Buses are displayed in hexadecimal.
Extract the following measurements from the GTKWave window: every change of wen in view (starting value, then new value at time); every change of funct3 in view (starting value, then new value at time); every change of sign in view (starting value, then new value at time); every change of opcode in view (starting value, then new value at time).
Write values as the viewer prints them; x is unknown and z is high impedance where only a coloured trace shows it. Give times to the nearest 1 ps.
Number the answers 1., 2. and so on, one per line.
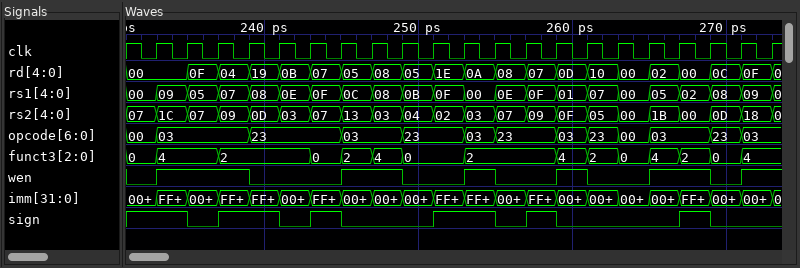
1. 0, 1 at 233 ps, 0 at 239 ps, 1 at 245 ps, 0 at 249 ps, 1 at 253 ps, 0 at 255 ps, 1 at 259 ps, 0 at 261 ps, 1 at 265 ps, 0 at 269 ps, 1 at 271 ps
2. 0, 4 at 233 ps, 2 at 237 ps, 0 at 243 ps, 2 at 245 ps, 4 at 247 ps, 0 at 249 ps, 2 at 253 ps, 4 at 259 ps, 2 at 261 ps, 0 at 263 ps, 4 at 265 ps, 2 at 267 ps, 0 at 269 ps, 4 at 271 ps
3. 1, 0 at 235 ps, 1 at 237 ps, 0 at 241 ps, 1 at 243 ps, 0 at 245 ps, 1 at 251 ps, 0 at 255 ps, 1 at 257 ps, 0 at 259 ps, 1 at 267 ps, 0 at 269 ps
4. 00, 03 at 233 ps, 23 at 239 ps, 03 at 245 ps, 23 at 249 ps, 03 at 253 ps, 23 at 255 ps, 03 at 259 ps, 23 at 261 ps, 00 at 263 ps, 03 at 265 ps, 23 at 269 ps, 03 at 271 ps
